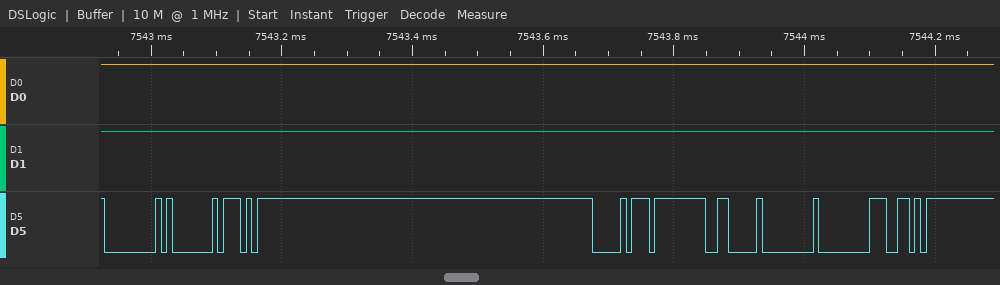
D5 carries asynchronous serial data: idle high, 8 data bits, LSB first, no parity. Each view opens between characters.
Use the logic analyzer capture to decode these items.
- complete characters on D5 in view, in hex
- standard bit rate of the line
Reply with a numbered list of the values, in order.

1. 00, 01, D7, D0, FF, 06, 00, 00, D6
2. 115200 baud
